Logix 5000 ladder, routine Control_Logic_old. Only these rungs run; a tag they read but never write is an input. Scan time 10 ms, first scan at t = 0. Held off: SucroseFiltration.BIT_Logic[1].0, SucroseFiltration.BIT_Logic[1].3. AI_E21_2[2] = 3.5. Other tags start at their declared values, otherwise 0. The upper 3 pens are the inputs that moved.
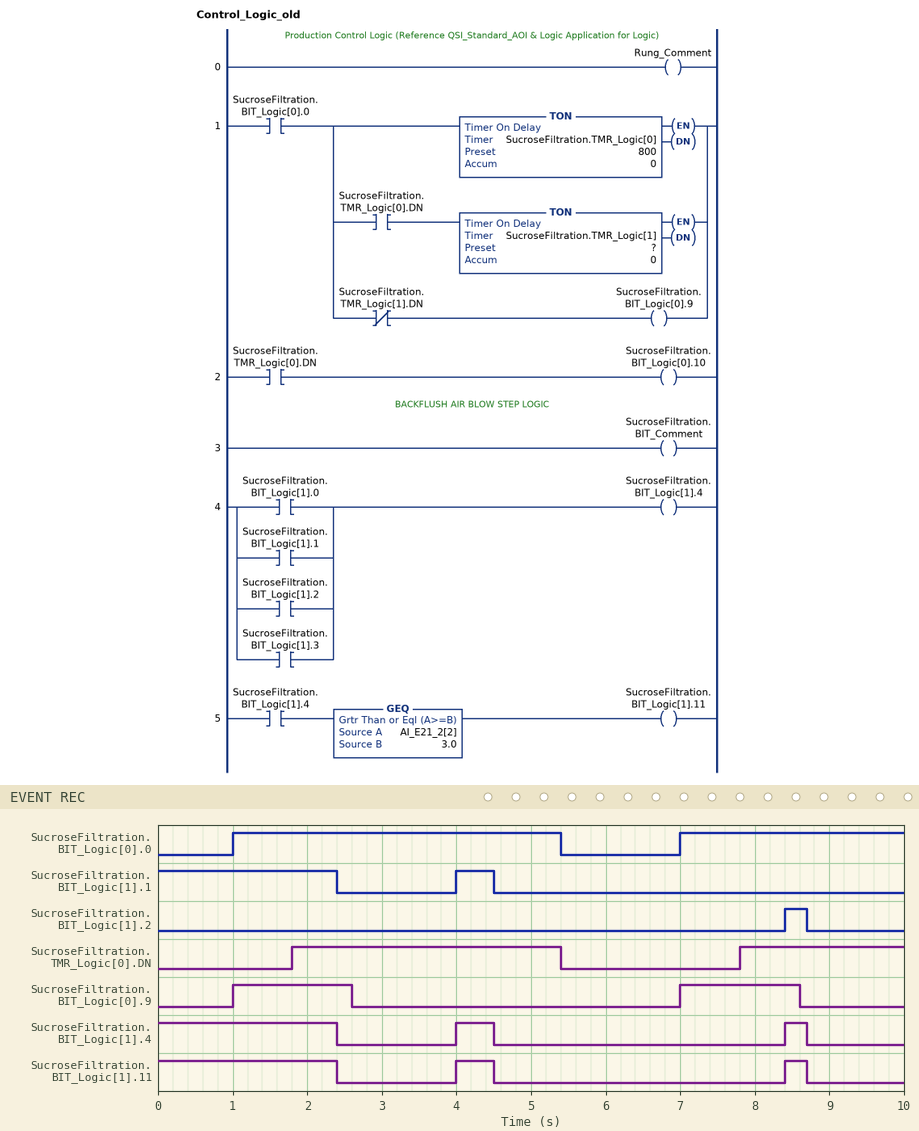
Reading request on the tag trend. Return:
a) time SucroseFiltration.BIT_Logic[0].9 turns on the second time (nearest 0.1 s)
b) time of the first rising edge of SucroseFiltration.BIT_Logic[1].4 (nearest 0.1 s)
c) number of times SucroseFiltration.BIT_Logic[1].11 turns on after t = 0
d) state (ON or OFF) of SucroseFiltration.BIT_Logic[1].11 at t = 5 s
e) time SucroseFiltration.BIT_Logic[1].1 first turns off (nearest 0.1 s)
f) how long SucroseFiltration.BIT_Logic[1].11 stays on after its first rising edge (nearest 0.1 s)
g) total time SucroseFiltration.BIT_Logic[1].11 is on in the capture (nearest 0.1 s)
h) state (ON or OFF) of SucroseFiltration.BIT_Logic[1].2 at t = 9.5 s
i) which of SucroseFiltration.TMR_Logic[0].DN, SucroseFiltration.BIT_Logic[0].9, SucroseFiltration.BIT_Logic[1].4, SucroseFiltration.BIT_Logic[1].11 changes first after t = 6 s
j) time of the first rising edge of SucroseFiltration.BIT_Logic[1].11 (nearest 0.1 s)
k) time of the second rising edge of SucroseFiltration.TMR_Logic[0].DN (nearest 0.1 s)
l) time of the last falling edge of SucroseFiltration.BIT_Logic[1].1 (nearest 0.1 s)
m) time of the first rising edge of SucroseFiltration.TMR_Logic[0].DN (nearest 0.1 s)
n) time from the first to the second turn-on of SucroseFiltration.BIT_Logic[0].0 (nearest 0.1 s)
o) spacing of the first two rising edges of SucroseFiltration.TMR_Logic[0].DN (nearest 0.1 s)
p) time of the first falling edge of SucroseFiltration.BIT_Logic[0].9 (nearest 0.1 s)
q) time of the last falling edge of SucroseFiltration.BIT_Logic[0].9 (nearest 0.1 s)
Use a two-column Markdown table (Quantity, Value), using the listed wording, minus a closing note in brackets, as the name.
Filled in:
| Quantity | Value |
|---|---|
| time SucroseFiltration.BIT_Logic[0].9 turns on the second time | 7.0 s |
| time of the first rising edge of SucroseFiltration.BIT_Logic[1].4 | 4.0 s |
| number of times SucroseFiltration.BIT_Logic[1].11 turns on after t = 0 | 2 |
| state (ON or OFF) of SucroseFiltration.BIT_Logic[1].11 at t = 5 s | OFF |
| time SucroseFiltration.BIT_Logic[1].1 first turns off | 2.4 s |
| how long SucroseFiltration.BIT_Logic[1].11 stays on after its first rising edge | 0.5 s |
| total time SucroseFiltration.BIT_Logic[1].11 is on in the capture | 3.2 s |
| state (ON or OFF) of SucroseFiltration.BIT_Logic[1].2 at t = 9.5 s | OFF |
| which of SucroseFiltration.TMR_Logic[0].DN, SucroseFiltration.BIT_Logic[0].9, SucroseFiltration.BIT_Logic[1].4, SucroseFiltration.BIT_Logic[1].11 changes first after t = 6 s | SucroseFiltration.BIT_Logic[0].9 |
| time of the first rising edge of SucroseFiltration.BIT_Logic[1].11 | 4.0 s |
| time of the second rising edge of SucroseFiltration.TMR_Logic[0].DN | 7.8 s |
| time of the last falling edge of SucroseFiltration.BIT_Logic[1].1 | 4.5 s |
| time of the first rising edge of SucroseFiltration.TMR_Logic[0].DN | 1.8 s |
| time from the first to the second turn-on of SucroseFiltration.BIT_Logic[0].0 | 6.0 s |
| spacing of the first two rising edges of SucroseFiltration.TMR_Logic[0].DN | 6.0 s |
| time of the first falling edge of SucroseFiltration.BIT_Logic[0].9 | 2.6 s |
| time of the last falling edge of SucroseFiltration.BIT_Logic[0].9 | 8.6 s |
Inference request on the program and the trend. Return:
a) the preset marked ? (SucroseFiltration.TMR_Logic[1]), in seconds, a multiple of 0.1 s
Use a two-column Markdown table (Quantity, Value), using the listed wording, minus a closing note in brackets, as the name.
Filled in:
| Quantity | Value |
|---|---|
| the preset marked ? (SucroseFiltration.TMR_Logic[1]), in seconds, a multiple of 0.1 s | 0.8 s |
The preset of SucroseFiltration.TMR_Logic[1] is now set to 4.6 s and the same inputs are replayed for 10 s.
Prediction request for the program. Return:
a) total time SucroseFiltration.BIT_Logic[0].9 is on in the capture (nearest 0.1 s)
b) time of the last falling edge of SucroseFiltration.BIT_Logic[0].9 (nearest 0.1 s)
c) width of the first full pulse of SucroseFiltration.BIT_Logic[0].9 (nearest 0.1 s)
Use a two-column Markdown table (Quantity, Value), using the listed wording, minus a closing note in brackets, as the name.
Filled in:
| Quantity | Value |
|---|---|
| total time SucroseFiltration.BIT_Logic[0].9 is on in the capture | 7.4 s |
| time of the last falling edge of SucroseFiltration.BIT_Logic[0].9 | 5.4 s |
| width of the first full pulse of SucroseFiltration.BIT_Logic[0].9 | 4.4 s |
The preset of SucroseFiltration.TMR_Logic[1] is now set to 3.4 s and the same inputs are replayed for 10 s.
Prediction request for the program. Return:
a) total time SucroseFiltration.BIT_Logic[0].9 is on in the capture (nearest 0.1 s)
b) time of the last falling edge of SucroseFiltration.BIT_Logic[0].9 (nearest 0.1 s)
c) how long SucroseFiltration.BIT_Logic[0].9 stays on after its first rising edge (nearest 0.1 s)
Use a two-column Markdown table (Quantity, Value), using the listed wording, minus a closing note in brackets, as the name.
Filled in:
| Quantity | Value |
|---|---|
| total time SucroseFiltration.BIT_Logic[0].9 is on in the capture | 7.2 s |
| time of the last falling edge of SucroseFiltration.BIT_Logic[0].9 | 5.2 s |
| how long SucroseFiltration.BIT_Logic[0].9 stays on after its first rising edge | 4.2 s |
